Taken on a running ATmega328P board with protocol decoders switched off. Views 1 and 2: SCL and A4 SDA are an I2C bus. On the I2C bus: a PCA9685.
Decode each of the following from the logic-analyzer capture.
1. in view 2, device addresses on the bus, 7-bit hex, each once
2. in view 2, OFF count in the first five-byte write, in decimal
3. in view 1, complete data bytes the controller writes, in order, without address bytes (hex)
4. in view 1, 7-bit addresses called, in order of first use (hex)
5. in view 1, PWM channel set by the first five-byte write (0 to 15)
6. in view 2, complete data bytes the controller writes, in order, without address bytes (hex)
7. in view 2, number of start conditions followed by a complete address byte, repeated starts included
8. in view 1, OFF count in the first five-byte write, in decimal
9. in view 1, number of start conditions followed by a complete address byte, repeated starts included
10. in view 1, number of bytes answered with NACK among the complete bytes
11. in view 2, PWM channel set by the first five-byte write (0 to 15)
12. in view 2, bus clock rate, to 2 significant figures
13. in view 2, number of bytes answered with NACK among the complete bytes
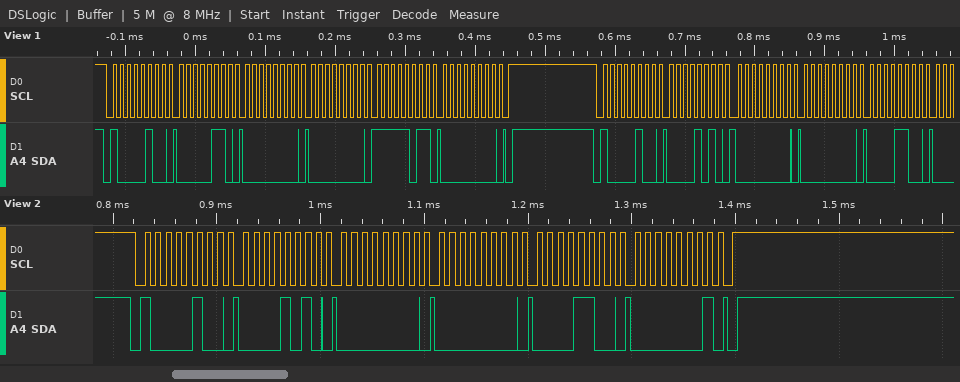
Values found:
0x42
268
06 00 00 FB 00 0A 00 00 0C
0x42
0
0A 00 00 0C 01
1
251
2
0
1
100 kHz
0
